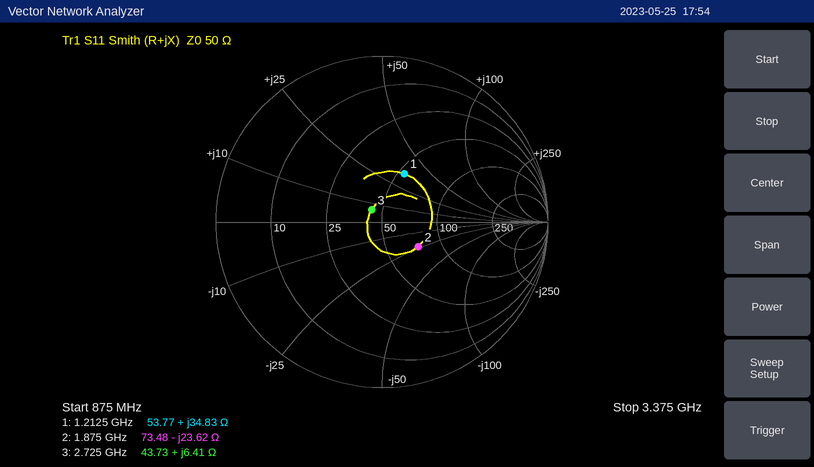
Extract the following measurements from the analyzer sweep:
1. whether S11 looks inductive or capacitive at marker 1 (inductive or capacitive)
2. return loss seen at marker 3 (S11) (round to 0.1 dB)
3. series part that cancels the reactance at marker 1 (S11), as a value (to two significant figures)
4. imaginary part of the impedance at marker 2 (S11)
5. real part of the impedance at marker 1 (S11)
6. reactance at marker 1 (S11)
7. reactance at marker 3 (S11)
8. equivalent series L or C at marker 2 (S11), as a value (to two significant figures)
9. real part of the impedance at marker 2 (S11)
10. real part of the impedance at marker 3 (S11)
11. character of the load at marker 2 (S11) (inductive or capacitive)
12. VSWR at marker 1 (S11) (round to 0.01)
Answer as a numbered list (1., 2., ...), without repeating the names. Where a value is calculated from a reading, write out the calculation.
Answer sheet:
1. inductive
2. 20.4 dB
3. C = 1/(2π × 1.2125 GHz × 34.83 Ω) ≈ 3.8 pF
4. -23.62 Ω
5. 53.77 Ω
6. +34.83 Ω
7. +6.41 Ω
8. C = 1/(2π × 1.875 GHz × 23.62 Ω) ≈ 3.6 pF
9. 73.48 Ω
10. 43.73 Ω
11. capacitive
12. 1.94
